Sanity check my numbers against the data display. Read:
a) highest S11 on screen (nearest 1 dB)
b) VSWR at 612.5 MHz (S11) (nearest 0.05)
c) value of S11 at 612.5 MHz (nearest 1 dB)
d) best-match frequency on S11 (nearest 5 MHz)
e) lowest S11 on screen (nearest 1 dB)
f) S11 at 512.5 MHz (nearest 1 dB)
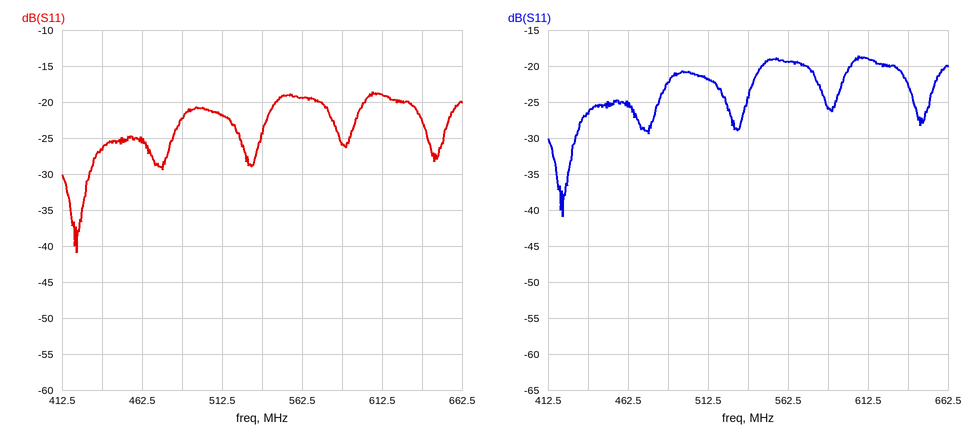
-19 dB
1.25
-19 dB
420 MHz
-41 dB
-22 dB
